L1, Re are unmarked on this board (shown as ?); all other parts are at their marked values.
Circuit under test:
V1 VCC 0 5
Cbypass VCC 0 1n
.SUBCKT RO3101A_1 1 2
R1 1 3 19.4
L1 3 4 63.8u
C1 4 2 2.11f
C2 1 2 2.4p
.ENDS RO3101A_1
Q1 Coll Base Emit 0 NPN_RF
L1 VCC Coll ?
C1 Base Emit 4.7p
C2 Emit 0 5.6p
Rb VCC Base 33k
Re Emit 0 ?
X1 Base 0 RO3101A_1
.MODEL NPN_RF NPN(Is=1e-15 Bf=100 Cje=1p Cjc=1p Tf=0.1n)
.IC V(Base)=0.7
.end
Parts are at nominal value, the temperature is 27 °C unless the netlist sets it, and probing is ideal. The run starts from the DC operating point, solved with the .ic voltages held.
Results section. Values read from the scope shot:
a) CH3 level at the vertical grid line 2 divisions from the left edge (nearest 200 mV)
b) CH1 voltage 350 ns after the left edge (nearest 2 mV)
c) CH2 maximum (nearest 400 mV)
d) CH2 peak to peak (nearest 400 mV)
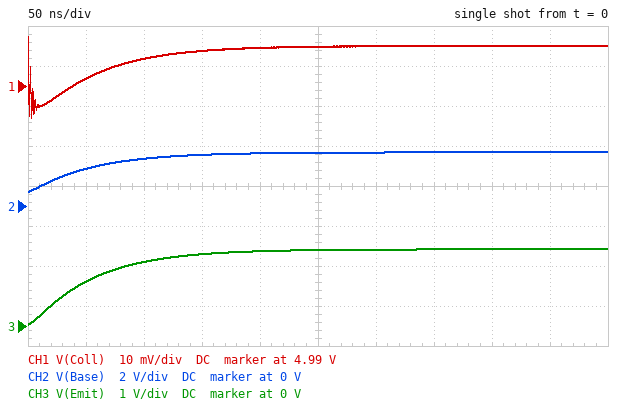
1.6 V
5.000 V
2.8 V
2.0 V
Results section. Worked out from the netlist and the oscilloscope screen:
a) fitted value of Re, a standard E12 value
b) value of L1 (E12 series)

270 Ω
150 nH
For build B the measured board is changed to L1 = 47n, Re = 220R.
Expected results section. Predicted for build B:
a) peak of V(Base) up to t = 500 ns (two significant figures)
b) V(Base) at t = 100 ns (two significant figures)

2.5 V
2.2 V
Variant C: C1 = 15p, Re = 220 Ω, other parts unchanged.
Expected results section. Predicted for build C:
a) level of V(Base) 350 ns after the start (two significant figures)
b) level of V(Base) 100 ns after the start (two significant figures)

2.5 V
2.2 V
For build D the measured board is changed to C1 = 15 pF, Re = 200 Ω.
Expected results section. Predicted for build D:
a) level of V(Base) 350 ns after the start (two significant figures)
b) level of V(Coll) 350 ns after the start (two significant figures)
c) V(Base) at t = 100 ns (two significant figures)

2.4 V
5.0 V
2.1 V
